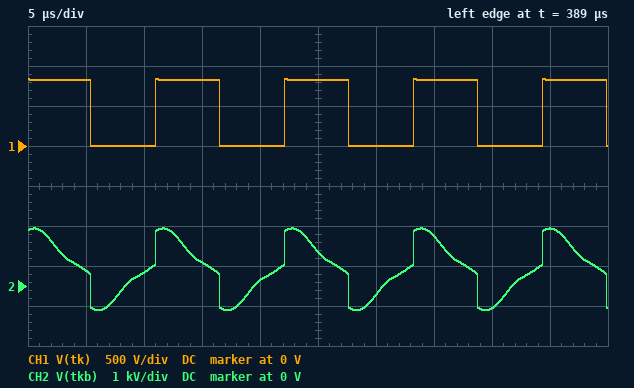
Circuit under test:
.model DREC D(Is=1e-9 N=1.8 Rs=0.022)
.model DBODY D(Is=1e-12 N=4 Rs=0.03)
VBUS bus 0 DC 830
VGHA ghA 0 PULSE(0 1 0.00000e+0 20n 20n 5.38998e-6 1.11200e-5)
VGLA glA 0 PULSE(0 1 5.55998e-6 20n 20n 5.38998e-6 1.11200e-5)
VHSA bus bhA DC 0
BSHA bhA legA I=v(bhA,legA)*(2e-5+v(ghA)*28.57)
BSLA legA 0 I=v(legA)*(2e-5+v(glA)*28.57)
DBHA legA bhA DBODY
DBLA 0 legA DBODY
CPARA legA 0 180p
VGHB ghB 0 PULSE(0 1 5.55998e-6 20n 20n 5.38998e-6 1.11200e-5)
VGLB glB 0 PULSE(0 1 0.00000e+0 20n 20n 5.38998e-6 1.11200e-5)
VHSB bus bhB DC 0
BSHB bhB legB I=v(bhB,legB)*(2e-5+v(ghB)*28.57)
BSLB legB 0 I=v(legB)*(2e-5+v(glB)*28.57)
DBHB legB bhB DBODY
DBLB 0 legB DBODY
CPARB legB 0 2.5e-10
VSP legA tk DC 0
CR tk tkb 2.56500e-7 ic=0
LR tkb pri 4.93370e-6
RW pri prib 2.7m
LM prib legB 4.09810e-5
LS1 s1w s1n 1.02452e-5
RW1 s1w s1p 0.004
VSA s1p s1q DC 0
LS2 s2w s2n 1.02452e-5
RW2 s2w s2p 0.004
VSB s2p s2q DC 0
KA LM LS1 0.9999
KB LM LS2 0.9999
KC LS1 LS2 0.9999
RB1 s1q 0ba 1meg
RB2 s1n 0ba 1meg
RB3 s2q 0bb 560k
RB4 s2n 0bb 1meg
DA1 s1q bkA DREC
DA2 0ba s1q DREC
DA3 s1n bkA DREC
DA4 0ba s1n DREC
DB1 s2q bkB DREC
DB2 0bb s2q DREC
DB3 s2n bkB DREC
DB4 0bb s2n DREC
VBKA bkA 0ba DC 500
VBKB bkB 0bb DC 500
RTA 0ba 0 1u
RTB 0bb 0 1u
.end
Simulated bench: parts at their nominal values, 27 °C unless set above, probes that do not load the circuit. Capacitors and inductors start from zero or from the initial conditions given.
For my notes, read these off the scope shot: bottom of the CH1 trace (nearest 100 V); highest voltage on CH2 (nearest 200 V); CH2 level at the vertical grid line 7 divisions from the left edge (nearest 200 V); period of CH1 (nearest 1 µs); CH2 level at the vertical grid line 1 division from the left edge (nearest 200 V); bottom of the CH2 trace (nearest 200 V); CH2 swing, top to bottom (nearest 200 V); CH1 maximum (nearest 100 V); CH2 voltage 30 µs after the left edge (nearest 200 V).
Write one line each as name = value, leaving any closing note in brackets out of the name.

bottom of the CH1 trace = 0 V
highest voltage on CH2 = 1.4 kV
CH2 level at the vertical grid line 7 divisions from the left edge = 1.2 kV
period of CH1 = 11 µs
CH2 level at the vertical grid line 1 division from the left edge = 400 V
bottom of the CH2 trace = -600 V
CH2 swing, top to bottom = 2.0 kV
CH1 maximum = 800 V
CH2 voltage 30 µs after the left edge = -200 V
